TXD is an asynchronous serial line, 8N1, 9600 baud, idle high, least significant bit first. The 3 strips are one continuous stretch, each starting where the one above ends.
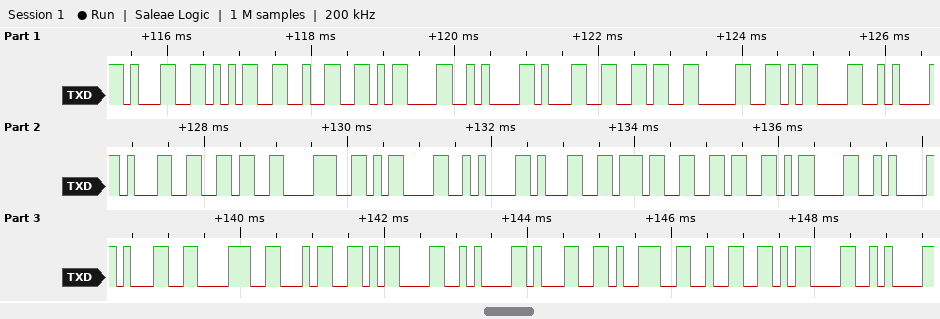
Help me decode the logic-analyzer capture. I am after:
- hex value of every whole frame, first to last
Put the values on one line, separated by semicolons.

31 35 32 0D 0A 31 36 30 0D 0A 31 36 38 0D 0A 31 37 36 0D 0A 31 38 34 0D 0A 31 39 32 0D 0A
